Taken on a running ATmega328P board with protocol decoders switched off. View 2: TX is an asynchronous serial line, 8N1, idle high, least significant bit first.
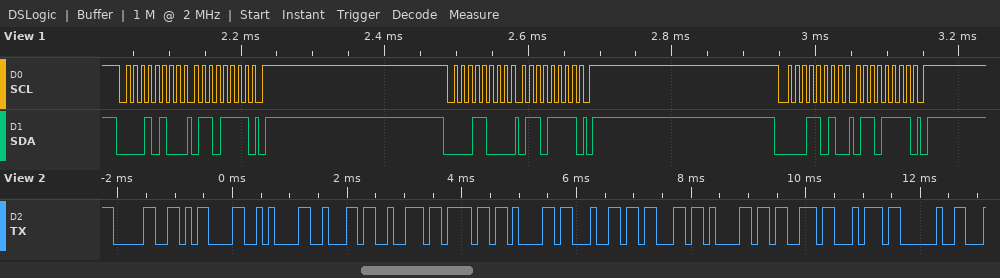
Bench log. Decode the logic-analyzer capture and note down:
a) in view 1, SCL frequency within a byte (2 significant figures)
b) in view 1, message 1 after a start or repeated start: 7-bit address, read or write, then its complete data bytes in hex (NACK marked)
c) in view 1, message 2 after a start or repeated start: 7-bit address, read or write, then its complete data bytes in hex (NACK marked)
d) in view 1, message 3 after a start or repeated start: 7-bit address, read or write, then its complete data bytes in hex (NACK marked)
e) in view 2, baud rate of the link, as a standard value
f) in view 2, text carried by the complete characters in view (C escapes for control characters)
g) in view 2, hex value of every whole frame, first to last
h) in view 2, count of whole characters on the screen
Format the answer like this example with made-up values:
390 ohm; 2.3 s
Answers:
100 kHz; 0x0A write: 6F; 0x0C write: 6F; 0x0D write: 6F; 9600 baud; "0\r\nbroadcast "; 30 0D 0A 62 72 6F 61 64 63 61 73 74 20; 13
